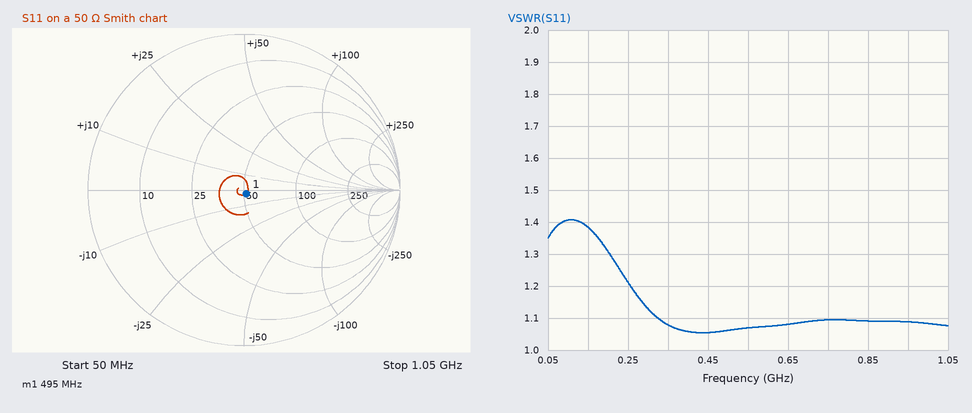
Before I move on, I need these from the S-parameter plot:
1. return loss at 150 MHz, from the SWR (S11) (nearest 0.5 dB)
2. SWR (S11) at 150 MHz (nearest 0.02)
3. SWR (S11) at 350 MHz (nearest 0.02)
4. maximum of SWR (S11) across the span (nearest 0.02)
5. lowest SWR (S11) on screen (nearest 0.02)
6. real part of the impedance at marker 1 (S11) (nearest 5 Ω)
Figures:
16.0 dB
1.38
1.08
1.40
1.06
50 Ω
